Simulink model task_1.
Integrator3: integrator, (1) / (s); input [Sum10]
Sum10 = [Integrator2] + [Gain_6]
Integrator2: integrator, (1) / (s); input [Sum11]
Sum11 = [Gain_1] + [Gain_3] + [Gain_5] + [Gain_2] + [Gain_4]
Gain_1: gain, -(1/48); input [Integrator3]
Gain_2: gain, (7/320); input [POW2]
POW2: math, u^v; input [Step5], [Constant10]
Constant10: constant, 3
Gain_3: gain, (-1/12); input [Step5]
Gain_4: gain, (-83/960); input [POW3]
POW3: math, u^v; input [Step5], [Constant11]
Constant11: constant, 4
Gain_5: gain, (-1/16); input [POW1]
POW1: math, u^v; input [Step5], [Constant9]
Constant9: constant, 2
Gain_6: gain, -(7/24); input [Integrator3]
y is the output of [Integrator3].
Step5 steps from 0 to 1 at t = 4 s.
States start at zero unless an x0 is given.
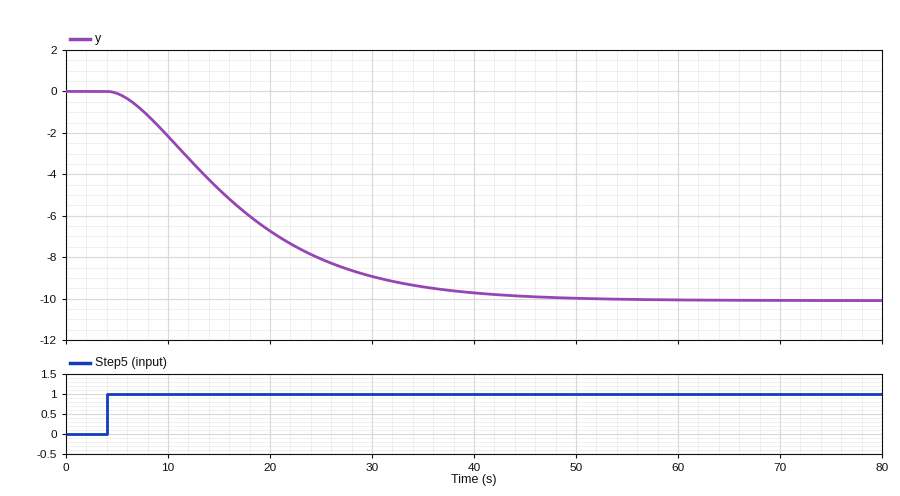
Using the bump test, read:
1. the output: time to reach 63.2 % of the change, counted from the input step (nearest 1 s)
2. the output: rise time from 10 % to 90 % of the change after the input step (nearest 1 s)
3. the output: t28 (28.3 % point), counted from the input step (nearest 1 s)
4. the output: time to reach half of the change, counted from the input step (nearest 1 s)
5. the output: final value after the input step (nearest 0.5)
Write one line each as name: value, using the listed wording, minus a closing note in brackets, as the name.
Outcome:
the output: time to reach 63.2 % of the change, counted from the input step: 15 s
the output: rise time from 10 % to 90 % of the change after the input step: 24 s
the output: t28 (28.3 % point), counted from the input step: 7 s
the output: time to reach half of the change, counted from the input step: 12 s
the output: final value after the input step: -10.0
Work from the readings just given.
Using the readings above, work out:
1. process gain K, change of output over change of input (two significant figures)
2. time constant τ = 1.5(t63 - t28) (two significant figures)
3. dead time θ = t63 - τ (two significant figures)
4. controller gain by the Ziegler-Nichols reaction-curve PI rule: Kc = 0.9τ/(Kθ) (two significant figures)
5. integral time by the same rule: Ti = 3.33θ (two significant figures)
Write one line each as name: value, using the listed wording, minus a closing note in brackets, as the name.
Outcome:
process gain K, change of output over change of input: -10
time constant τ = 1.5(t63 - t28): 12 s
dead time θ = t63 - τ: 3.0 s
controller gain by the Ziegler-Nichols reaction-curve PI rule: Kc = 0.9τ/(Kθ): -0.36
integral time by the same rule: Ti = 3.33θ: 10.0 s
